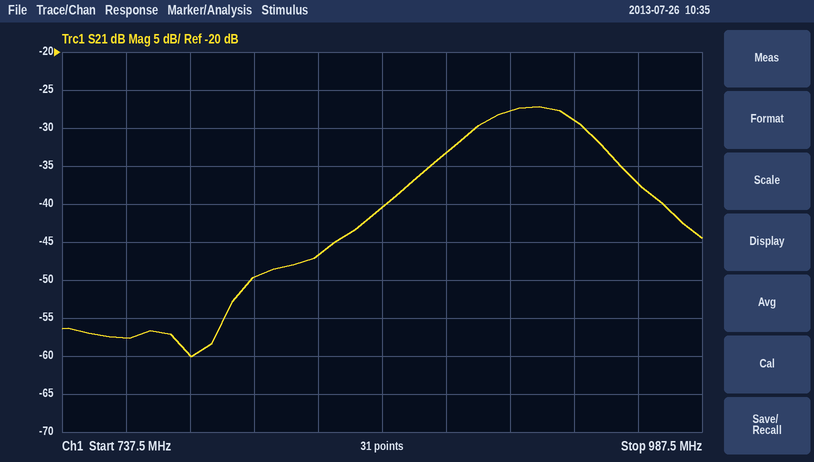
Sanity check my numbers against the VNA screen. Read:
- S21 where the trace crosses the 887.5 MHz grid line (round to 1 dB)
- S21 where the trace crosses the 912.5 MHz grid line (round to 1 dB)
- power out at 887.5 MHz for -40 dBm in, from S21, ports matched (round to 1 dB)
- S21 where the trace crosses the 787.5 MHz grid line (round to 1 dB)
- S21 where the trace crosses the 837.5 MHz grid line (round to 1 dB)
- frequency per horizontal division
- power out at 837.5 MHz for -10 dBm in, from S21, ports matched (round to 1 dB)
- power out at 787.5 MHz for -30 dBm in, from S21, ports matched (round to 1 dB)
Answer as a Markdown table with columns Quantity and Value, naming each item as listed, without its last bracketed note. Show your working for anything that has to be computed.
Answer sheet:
| Quantity | Value |
|---|---|
| S21 where the trace crosses the 887.5 MHz grid line | -33 dB |
| S21 where the trace crosses the 912.5 MHz grid line | -28 dB |
| power out at 887.5 MHz for -40 dBm in, from S21, ports matched | -40 dBm + (-33 dB) = -73 dBm |
| S21 where the trace crosses the 787.5 MHz grid line | -60 dB |
| S21 where the trace crosses the 837.5 MHz grid line | -47 dB |
| frequency per horizontal division | 25 MHz |
| power out at 837.5 MHz for -10 dBm in, from S21, ports matched | -10 dBm + (-47 dB) = -57 dBm |
| power out at 787.5 MHz for -30 dBm in, from S21, ports matched | -30 dBm + (-60 dB) = -90 dBm |
